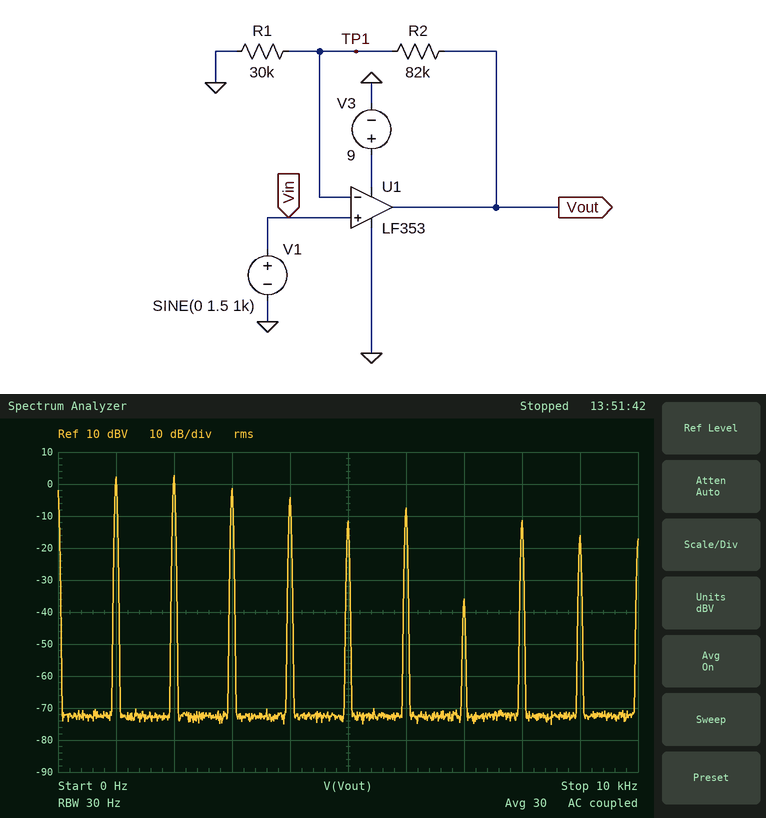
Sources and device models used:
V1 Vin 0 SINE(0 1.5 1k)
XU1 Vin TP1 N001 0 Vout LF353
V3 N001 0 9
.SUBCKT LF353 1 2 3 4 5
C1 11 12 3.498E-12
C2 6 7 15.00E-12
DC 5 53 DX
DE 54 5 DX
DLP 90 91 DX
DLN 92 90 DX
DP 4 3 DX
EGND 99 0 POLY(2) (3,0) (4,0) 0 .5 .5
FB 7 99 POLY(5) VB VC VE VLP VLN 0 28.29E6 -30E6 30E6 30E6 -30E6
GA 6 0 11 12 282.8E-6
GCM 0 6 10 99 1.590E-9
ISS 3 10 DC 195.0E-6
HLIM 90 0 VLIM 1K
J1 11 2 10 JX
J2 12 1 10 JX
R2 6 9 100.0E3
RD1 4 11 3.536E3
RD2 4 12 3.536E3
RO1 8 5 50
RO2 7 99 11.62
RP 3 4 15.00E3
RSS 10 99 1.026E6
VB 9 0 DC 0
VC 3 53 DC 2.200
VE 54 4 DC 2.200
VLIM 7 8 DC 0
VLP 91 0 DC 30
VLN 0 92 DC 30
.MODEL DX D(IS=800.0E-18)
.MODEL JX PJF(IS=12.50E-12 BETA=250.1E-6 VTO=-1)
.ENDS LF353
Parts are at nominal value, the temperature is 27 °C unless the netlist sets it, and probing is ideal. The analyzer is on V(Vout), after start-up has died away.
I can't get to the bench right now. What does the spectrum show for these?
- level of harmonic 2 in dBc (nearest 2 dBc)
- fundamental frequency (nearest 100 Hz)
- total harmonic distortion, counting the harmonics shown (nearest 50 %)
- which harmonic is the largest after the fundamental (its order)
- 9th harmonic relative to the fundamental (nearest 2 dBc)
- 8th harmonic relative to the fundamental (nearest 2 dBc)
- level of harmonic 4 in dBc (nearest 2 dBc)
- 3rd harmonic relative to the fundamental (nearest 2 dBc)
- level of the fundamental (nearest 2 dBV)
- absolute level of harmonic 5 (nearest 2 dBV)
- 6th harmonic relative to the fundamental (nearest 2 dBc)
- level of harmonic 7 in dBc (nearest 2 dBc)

0 dBc
1.0 kHz
150 %
2
-18 dBc
-14 dBc
-6 dBc
-4 dBc
2 dBV
-12 dBV
-10 dBc
-38 dBc
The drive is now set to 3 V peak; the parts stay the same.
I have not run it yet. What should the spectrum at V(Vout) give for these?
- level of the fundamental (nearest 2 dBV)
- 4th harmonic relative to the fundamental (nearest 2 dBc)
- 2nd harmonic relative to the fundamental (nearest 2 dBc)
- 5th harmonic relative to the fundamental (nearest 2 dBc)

-12 dBV
10 dBc
14 dBc
8 dBc
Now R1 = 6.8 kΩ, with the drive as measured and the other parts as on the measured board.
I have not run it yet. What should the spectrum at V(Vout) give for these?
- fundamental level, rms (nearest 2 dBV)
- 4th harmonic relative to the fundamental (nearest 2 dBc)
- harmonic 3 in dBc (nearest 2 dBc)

-24 dBV
24 dBc
4 dBc
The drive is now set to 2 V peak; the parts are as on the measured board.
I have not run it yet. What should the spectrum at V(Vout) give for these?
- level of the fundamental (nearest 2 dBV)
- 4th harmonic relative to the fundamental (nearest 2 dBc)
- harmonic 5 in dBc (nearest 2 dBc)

-4 dBV
-2 dBc
-4 dBc
